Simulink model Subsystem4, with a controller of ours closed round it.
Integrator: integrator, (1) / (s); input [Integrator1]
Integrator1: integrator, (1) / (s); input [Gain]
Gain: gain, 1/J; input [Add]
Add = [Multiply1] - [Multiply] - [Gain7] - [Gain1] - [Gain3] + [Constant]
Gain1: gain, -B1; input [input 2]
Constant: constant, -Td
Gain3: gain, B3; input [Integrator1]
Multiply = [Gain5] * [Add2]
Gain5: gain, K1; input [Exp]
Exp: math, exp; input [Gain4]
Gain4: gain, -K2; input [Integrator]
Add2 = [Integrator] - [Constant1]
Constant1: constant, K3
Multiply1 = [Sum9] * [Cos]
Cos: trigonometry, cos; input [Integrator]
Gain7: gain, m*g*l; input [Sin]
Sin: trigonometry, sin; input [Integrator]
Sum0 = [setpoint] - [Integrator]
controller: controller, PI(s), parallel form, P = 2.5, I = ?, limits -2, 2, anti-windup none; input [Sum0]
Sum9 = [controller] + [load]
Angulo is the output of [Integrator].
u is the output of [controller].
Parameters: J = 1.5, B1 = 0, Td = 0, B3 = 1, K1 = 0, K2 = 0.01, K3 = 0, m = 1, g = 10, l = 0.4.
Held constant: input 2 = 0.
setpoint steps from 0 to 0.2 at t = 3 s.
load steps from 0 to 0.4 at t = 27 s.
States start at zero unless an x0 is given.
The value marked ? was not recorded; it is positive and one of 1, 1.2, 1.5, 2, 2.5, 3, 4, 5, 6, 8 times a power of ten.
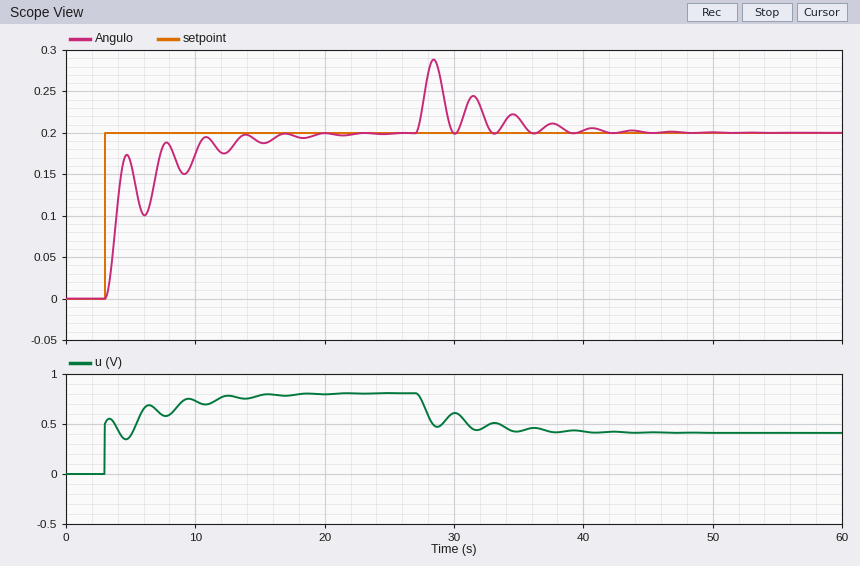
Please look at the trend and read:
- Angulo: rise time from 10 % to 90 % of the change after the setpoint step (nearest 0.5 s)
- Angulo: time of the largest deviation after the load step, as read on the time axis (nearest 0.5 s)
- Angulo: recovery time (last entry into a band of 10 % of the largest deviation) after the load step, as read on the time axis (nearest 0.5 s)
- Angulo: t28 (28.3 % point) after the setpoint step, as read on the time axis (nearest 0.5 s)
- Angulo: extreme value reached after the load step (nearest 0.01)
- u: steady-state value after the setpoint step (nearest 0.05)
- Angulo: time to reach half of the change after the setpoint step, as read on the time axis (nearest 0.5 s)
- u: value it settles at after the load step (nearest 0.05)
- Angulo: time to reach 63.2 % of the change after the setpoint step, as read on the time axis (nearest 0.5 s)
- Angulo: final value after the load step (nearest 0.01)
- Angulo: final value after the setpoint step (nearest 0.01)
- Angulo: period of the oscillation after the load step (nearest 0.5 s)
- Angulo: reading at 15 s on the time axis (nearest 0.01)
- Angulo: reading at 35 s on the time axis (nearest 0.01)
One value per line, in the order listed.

4.0 s
28.5 s
38.0 s
3.5 s
0.29
0.80
4.0 s
0.40
4.0 s
0.20
0.20
3.0 s
0.19
0.22
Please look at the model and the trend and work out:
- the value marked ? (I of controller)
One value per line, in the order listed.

1.5
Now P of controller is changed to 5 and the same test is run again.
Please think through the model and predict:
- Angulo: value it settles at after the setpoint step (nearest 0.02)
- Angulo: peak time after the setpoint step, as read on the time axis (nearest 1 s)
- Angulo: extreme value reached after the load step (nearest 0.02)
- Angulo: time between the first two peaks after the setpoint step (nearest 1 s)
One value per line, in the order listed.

0.20
4 s
0.26
3 s
